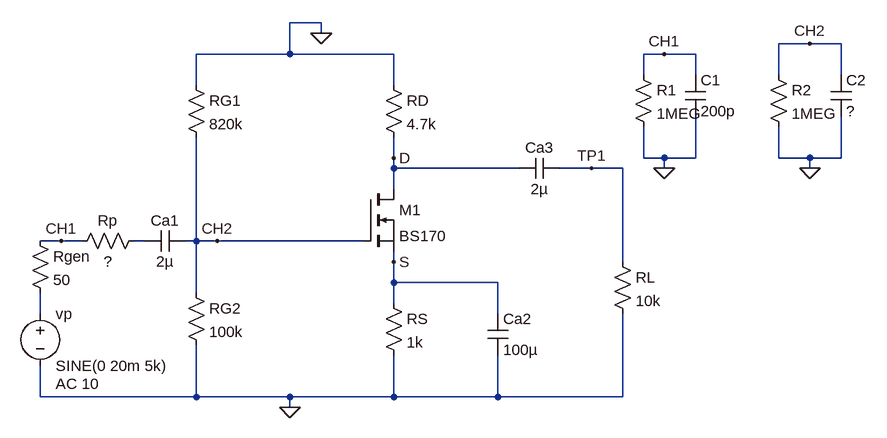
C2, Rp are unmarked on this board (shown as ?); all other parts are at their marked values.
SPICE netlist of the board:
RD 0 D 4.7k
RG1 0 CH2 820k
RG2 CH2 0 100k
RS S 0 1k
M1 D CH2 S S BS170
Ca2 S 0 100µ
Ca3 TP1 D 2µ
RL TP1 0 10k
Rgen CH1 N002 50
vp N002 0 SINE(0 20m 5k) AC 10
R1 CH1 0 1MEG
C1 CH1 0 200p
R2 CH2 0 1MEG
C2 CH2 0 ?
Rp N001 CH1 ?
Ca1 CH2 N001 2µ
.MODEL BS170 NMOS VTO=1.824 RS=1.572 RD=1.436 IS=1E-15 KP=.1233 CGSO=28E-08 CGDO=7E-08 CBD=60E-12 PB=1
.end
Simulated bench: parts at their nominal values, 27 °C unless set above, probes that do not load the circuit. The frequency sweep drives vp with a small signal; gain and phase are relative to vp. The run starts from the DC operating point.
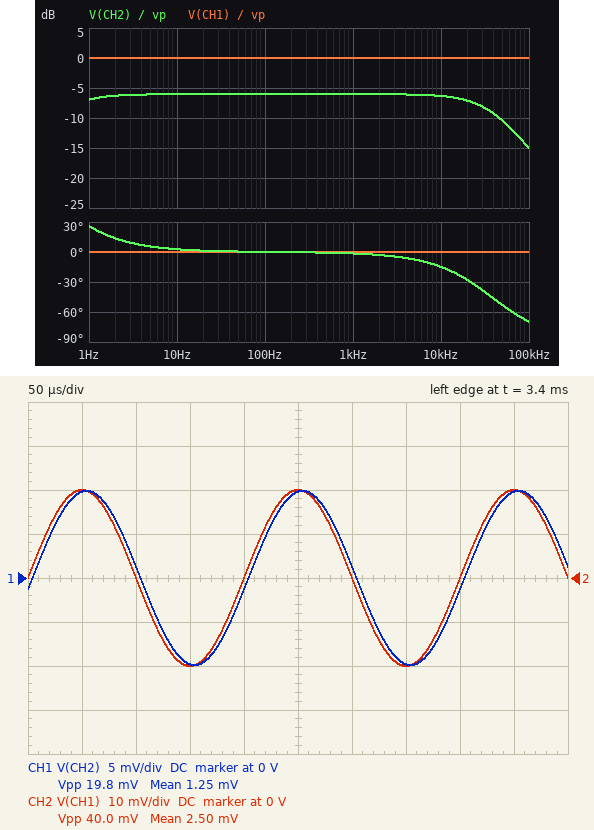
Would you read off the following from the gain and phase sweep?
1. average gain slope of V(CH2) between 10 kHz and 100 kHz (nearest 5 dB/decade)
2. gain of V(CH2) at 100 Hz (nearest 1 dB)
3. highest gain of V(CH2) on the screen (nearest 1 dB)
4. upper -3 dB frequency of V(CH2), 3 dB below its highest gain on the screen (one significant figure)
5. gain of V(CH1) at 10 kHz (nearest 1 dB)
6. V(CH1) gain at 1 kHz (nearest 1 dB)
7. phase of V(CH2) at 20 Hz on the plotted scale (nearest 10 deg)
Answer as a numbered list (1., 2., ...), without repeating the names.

1. -10 dB/decade
2. -6 dB
3. -6 dB
4. 40 kHz
5. 0 dB
6. 0 dB
7. 0 deg
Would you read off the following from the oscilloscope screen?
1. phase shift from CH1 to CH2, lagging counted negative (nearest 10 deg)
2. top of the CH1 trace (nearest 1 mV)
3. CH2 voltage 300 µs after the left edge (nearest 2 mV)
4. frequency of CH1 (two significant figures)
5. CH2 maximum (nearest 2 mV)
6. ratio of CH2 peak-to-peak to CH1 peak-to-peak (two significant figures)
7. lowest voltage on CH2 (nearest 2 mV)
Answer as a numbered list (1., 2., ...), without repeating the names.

1. 10 deg
2. 10 mV
3. 0 V
4. 5.0 kHz
5. 20 mV
6. 2.0
7. -20 mV
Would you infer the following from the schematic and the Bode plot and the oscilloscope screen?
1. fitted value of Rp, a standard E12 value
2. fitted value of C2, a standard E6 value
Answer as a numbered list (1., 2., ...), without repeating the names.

1. 82 kΩ
2. 68 pF
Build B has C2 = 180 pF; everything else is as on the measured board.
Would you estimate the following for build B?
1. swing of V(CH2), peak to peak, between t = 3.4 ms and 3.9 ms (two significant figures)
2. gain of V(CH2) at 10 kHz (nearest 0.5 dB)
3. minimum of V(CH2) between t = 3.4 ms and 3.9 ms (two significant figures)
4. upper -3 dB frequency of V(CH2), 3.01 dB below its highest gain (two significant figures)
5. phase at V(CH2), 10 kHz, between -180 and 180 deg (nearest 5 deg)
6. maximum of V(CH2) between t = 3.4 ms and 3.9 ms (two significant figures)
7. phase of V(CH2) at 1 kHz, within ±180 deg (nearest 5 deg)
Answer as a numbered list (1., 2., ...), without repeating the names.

1. 19 mV
2. -7.0 dB
3. -9.6 mV
4. 18 kHz
5. -30 deg
6. 9.6 mV
7. -5 deg
